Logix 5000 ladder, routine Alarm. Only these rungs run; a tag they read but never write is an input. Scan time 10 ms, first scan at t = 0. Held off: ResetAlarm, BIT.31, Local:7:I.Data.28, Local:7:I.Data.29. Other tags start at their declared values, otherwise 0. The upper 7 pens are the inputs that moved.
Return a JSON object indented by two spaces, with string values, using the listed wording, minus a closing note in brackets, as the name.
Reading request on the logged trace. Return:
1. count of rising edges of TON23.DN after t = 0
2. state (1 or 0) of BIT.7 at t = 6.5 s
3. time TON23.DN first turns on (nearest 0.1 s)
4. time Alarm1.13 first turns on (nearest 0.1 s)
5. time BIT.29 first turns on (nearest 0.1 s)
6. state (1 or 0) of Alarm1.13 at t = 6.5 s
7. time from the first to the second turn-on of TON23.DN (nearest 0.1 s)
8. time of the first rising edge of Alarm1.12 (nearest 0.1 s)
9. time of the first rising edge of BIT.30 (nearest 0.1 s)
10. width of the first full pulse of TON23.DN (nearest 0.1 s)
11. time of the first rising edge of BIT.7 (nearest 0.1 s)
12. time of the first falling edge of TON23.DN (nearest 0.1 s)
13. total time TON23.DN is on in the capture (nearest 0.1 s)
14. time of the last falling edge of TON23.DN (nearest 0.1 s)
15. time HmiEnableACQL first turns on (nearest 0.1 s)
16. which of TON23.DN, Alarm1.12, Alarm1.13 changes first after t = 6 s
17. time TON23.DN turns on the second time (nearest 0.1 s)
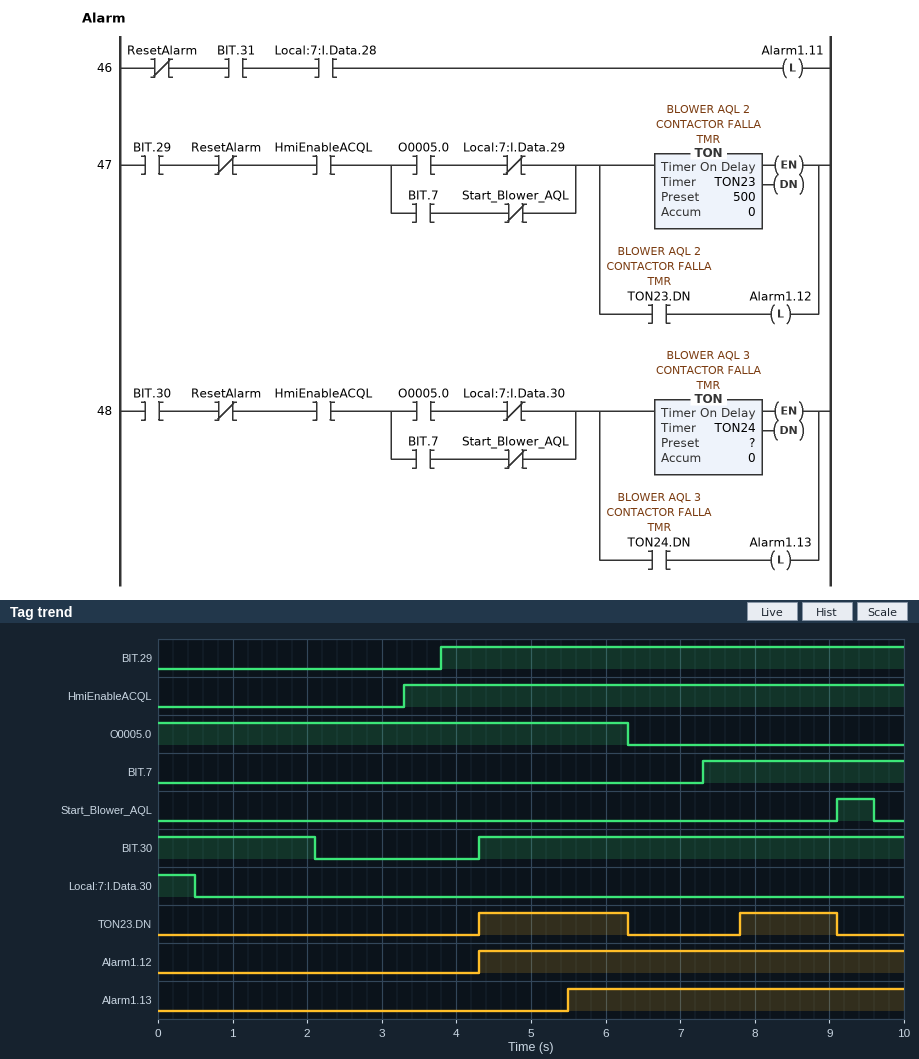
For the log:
{
  "count of rising edges of TON23.DN after t = 0": "2",
  "state (1 or 0) of BIT.7 at t = 6.5 s": "0",
  "time TON23.DN first turns on": "4.3 s",
  "time Alarm1.13 first turns on": "5.5 s",
  "time BIT.29 first turns on": "3.8 s",
  "state (1 or 0) of Alarm1.13 at t = 6.5 s": "1",
  "time from the first to the second turn-on of TON23.DN": "3.5 s",
  "time of the first rising edge of Alarm1.12": "4.3 s",
  "time of the first rising edge of BIT.30": "4.3 s",
  "width of the first full pulse of TON23.DN": "2.0 s",
  "time of the first rising edge of BIT.7": "7.3 s",
  "time of the first falling edge of TON23.DN": "6.3 s",
  "total time TON23.DN is on in the capture": "3.3 s",
  "time of the last falling edge of TON23.DN": "9.1 s",
  "time HmiEnableACQL first turns on": "3.3 s",
  "which of TON23.DN, Alarm1.12, Alarm1.13 changes first after t = 6 s": "TON23.DN",
  "time TON23.DN turns on the second time": "7.8 s"
}
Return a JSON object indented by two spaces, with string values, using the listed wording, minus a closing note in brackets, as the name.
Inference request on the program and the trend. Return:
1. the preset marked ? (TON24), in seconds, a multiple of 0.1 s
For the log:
{
  "the preset marked ? (TON24), in seconds, a multiple of 0.1 s": "1.2 s"
}
